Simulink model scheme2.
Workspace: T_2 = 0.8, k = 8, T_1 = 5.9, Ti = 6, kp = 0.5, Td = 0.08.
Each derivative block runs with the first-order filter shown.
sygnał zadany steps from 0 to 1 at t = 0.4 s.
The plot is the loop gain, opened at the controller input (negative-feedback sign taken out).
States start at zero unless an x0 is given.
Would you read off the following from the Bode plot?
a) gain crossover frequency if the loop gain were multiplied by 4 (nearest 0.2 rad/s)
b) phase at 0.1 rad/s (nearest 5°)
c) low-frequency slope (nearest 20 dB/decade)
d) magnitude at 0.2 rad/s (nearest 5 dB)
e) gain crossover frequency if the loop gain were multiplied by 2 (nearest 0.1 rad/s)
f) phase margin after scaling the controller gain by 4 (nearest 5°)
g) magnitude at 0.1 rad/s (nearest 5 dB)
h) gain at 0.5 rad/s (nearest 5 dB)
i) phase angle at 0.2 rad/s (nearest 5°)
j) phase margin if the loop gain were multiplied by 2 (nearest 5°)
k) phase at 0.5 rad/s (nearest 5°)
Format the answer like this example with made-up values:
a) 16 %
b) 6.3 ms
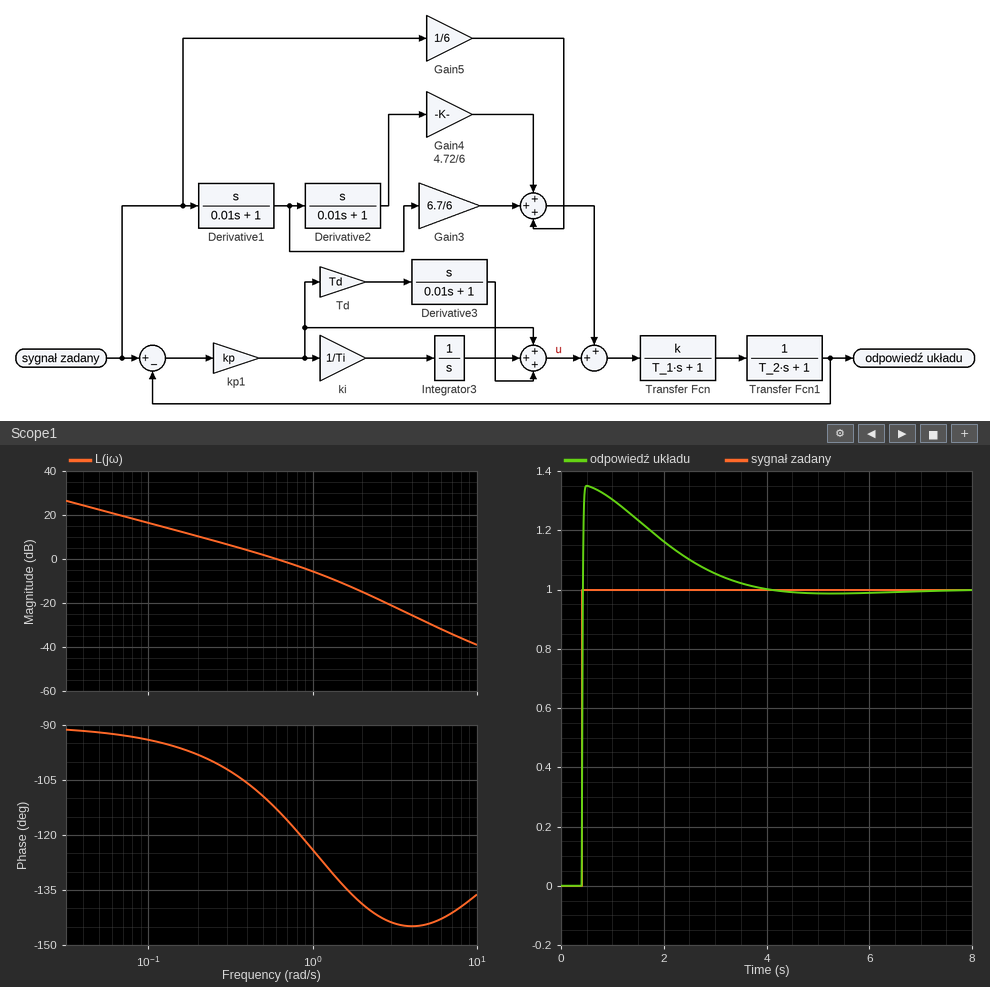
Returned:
a) 1.6 rad/s
b) -95°
c) -20 dB/decade
d) 10 dB
e) 1.0 rad/s
f) 45°
g) 15 dB
h) 0 dB
i) -100°
j) 55°
k) -110°
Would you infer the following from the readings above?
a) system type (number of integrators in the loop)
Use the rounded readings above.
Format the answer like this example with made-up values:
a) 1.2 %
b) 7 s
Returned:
a) 1
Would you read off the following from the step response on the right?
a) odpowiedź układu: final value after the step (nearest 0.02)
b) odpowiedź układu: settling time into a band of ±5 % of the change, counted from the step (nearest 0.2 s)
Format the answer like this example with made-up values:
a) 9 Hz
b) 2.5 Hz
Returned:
a) 1.00
b) 2.6 s
